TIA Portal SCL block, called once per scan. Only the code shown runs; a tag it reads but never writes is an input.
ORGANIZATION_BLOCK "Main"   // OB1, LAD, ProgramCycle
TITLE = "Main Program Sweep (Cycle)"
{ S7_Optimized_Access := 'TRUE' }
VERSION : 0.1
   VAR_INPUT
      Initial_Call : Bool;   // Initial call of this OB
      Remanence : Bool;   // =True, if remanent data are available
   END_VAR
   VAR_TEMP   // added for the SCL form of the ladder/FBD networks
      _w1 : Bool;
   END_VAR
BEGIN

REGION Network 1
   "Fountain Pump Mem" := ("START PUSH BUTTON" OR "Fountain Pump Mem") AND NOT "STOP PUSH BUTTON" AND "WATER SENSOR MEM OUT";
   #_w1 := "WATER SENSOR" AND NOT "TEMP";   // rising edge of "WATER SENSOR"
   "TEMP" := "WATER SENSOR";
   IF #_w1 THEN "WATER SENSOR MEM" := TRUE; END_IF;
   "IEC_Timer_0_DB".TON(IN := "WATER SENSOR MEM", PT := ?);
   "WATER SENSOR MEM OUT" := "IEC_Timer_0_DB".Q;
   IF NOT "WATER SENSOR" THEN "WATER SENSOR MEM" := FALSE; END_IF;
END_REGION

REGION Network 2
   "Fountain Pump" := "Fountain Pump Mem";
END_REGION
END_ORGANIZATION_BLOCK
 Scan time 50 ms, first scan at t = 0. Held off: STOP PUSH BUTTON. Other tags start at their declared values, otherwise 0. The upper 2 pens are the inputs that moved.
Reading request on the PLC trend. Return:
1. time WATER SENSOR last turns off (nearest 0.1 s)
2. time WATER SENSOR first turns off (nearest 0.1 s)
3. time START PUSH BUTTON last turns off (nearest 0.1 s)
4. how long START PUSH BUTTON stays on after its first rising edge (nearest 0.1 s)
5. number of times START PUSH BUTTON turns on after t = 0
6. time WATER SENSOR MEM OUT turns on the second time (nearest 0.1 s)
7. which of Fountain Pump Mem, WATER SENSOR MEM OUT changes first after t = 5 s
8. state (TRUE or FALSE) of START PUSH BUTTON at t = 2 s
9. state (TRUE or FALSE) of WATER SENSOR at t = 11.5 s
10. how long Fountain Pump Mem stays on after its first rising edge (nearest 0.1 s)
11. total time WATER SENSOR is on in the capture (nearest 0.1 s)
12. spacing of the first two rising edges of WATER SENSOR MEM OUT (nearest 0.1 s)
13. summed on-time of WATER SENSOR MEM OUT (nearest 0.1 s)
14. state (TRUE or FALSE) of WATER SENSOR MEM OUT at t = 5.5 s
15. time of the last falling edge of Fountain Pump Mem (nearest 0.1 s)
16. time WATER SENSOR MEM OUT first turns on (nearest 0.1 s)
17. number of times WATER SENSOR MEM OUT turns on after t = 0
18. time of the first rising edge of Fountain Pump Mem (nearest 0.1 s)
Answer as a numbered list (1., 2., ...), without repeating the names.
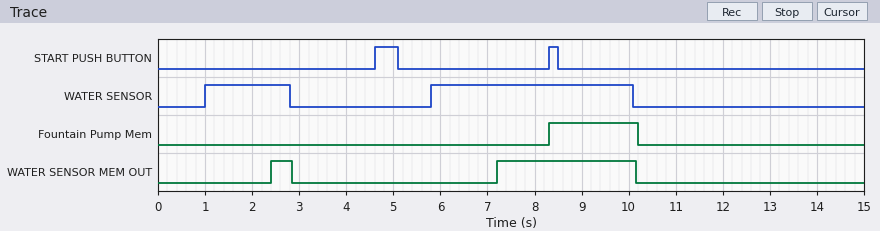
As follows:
1. 10.1 s
2. 2.8 s
3. 8.5 s
4. 0.5 s
5. 2
6. 7.2 s
7. WATER SENSOR MEM OUT
8. FALSE
9. FALSE
10. 1.9 s
11. 6.1 s
12. 4.8 s
13. 3.4 s
14. FALSE
15. 10.2 s
16. 2.4 s
17. 2
18. 8.3 s
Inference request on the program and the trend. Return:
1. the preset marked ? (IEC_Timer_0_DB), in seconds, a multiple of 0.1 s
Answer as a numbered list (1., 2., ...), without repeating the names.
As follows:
1. 1.4 s
